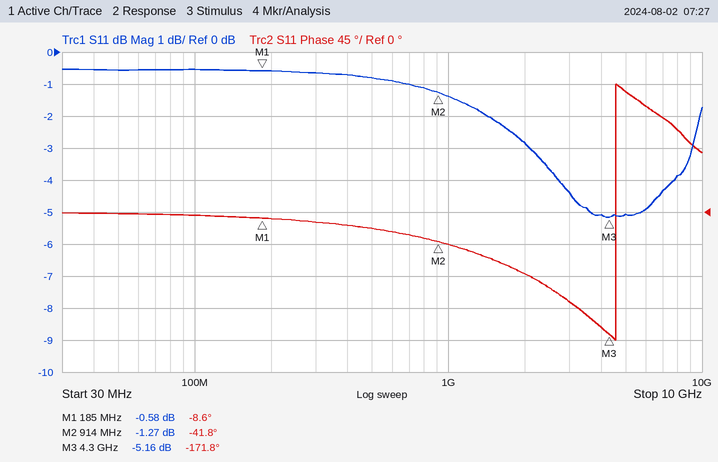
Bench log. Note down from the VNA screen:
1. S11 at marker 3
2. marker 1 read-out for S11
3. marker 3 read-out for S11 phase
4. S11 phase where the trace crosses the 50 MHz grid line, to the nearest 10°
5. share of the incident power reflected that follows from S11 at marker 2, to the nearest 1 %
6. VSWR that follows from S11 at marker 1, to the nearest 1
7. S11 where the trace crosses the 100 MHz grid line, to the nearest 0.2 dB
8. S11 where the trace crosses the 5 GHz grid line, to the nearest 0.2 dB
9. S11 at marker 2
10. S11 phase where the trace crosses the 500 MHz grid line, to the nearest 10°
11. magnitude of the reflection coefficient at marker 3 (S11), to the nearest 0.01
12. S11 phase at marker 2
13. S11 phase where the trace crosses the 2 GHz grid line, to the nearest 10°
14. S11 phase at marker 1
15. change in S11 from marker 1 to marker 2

-5.16 dB
-0.58 dB
-171.8°
0°
75 %
30
-0.6 dB
-5.0 dB
-1.27 dB
-20°
0.55
-41.8°
-90°
-8.6°
-0.69 dB
